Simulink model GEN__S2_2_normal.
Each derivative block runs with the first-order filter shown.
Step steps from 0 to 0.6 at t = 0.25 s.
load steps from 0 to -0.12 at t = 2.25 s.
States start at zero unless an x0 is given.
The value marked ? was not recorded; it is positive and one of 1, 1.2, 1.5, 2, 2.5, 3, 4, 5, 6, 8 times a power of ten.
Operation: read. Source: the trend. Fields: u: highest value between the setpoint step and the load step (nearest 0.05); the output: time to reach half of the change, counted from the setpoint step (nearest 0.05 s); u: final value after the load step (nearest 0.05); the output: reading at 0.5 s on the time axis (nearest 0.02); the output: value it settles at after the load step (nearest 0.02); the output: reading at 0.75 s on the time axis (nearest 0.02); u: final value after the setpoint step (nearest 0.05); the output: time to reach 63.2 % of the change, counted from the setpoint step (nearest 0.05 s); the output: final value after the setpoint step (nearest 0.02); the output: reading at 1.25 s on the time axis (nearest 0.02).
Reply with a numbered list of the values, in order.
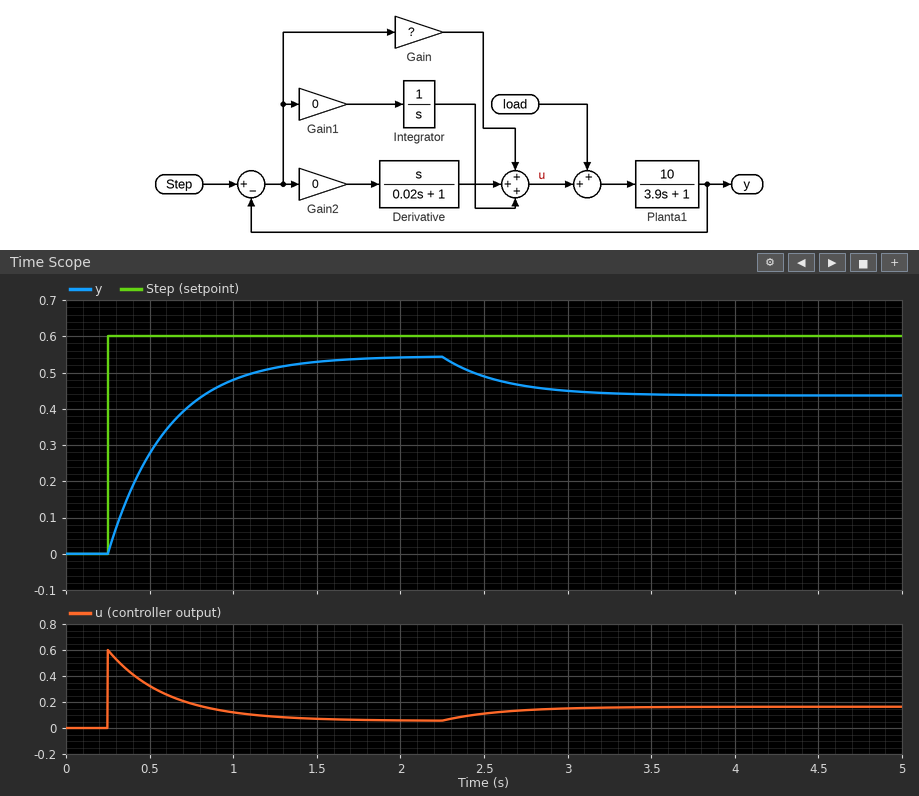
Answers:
1. 0.60
2. 0.25 s
3. 0.15
4. 0.28
5. 0.44
6. 0.42
7. 0.05
8. 0.35 s
9. 0.54
10. 0.52
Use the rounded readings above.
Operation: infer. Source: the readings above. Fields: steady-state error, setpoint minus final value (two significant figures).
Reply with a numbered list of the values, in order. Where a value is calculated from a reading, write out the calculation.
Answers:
1. 0.6 - 0.54 = 0.060
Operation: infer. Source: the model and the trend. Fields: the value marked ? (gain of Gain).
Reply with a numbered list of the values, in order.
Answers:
1. 1
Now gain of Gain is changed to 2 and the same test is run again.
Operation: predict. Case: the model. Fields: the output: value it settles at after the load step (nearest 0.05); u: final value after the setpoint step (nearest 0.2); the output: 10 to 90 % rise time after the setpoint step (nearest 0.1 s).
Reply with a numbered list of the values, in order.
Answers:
1. 0.50
2. 0.0
3. 0.4 s
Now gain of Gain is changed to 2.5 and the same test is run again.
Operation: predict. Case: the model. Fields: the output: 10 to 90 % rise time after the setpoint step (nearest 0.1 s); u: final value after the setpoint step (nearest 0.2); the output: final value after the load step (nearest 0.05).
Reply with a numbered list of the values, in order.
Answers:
1. 0.3 s
2. 0.0
3. 0.55
